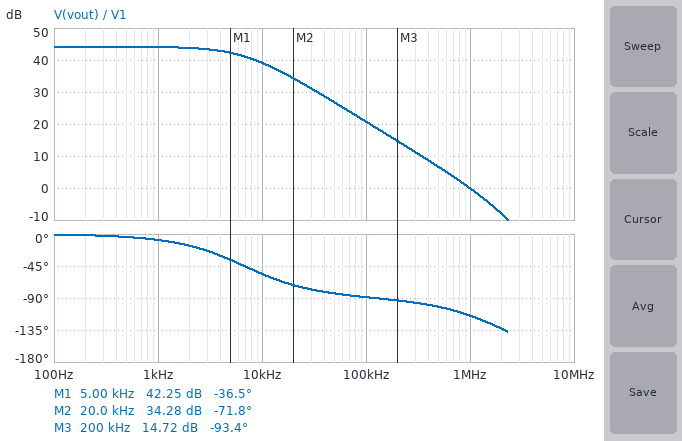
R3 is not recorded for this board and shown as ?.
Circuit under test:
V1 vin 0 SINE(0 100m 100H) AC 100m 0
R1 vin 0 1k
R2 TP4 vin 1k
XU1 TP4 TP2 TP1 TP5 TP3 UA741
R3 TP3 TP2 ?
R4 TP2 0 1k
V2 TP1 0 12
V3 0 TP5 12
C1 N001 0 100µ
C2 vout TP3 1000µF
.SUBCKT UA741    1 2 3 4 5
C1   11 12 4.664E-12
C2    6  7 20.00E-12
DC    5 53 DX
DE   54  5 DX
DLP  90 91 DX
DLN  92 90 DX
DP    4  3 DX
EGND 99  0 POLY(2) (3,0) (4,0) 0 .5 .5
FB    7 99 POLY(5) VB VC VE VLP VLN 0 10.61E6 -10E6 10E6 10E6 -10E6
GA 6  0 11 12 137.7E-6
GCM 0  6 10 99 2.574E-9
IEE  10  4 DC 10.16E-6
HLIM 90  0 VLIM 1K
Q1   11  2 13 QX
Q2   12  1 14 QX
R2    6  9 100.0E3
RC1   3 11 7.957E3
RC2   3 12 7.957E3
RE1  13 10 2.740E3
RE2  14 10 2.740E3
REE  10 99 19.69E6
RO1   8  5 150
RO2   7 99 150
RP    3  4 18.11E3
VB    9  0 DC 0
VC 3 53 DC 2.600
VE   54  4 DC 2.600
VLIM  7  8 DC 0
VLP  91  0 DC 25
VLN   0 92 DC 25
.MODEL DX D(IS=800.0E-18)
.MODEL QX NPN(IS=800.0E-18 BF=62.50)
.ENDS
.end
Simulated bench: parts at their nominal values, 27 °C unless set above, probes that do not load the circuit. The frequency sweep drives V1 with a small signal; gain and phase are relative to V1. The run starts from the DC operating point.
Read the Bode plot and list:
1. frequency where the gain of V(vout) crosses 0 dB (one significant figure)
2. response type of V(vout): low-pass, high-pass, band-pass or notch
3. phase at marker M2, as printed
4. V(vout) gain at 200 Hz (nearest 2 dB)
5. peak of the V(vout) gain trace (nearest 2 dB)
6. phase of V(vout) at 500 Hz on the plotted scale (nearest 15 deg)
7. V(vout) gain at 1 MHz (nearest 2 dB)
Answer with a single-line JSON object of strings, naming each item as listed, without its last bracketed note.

{"frequency where the gain of V(vout) crosses 0 dB": "1 MHz", "response type of V(vout): low-pass, high-pass, band-pass or notch": "low-pass", "phase at marker M2, as printed": "-71.8 deg", "V(vout) gain at 200 Hz": "44 dB", "peak of the V(vout) gain trace": "44 dB", "phase of V(vout) at 500 Hz on the plotted scale": "0 deg", "V(vout) gain at 1 MHz": "0 dB"}
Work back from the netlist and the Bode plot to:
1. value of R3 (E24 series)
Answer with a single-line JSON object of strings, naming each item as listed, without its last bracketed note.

{"value of R3": "160 kΩ"}
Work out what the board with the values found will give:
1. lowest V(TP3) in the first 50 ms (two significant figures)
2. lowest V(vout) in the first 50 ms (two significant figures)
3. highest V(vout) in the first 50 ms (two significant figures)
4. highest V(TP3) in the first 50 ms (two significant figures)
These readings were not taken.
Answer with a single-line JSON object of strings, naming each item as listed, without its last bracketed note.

{"lowest V(TP3) in the first 50 ms": "-10 V", "lowest V(vout) in the first 50 ms": "-10 V", "highest V(vout) in the first 50 ms": "10 V", "highest V(TP3) in the first 50 ms": "10 V"}
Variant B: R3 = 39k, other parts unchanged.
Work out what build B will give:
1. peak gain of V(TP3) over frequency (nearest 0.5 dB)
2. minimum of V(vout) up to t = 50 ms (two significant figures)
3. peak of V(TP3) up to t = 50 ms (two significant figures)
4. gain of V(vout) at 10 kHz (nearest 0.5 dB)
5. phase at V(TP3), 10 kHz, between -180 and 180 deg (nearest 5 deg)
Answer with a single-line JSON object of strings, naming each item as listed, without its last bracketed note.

{"peak gain of V(TP3) over frequency": "32.0 dB", "minimum of V(vout) up to t = 50 ms": "-4.0 V", "peak of V(TP3) up to t = 50 ms": "4.0 V", "gain of V(vout) at 10 kHz": "31.5 dB", "phase at V(TP3), 10 kHz, between -180 and 180 deg": "-20 deg"}
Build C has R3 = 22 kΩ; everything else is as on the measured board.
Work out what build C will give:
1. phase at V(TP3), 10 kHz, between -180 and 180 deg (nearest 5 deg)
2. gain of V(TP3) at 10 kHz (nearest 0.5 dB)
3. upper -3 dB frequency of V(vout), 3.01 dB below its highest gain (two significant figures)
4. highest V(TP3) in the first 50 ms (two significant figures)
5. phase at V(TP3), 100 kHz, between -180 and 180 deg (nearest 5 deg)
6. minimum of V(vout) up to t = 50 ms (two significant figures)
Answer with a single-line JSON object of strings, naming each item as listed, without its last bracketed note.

{"phase at V(TP3), 10 kHz, between -180 and 180 deg": "-10 deg", "gain of V(TP3) at 10 kHz": "27.0 dB", "upper -3 dB frequency of V(vout), 3.01 dB below its highest gain": "48 kHz", "highest V(TP3) in the first 50 ms": "2.3 V", "phase at V(TP3), 100 kHz, between -180 and 180 deg": "-65 deg", "minimum of V(vout) up to t = 50 ms": "-2.3 V"}
